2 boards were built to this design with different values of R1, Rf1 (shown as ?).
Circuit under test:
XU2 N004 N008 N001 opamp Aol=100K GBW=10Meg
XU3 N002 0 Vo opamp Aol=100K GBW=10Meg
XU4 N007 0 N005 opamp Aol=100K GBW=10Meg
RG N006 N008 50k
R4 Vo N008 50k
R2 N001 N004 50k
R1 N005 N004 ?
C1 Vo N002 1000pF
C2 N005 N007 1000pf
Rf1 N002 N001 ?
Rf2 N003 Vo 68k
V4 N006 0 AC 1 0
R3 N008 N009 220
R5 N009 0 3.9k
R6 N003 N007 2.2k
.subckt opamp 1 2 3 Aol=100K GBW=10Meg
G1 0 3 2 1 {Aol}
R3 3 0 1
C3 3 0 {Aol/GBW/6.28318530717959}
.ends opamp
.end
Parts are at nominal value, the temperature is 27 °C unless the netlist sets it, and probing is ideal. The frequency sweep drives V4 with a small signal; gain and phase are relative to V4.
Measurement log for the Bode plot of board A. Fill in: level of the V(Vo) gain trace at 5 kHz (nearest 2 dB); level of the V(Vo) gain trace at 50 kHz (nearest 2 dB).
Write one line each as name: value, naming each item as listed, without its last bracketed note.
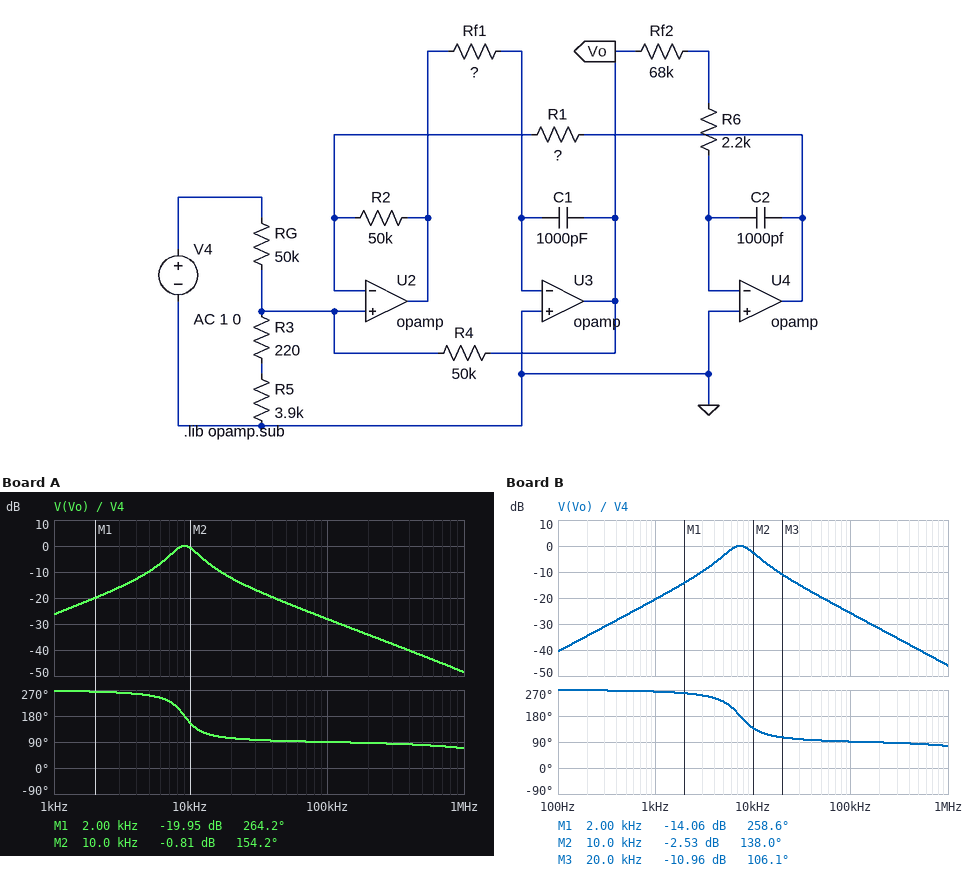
level of the V(Vo) gain trace at 5 kHz: -10 dB
level of the V(Vo) gain trace at 50 kHz: -22 dB
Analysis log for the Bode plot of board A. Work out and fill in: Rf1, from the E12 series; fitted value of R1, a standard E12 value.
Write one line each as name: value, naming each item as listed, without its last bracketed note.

Rf1, from the E12 series: 8.2 kΩ
fitted value of R1, a standard E12 value: 27 kΩ
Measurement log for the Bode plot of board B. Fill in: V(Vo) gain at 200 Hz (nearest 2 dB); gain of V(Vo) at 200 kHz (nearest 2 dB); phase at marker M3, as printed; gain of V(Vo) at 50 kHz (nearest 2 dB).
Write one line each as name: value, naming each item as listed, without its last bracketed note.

V(Vo) gain at 200 Hz: -34 dB
gain of V(Vo) at 200 kHz: -32 dB
phase at marker M3, as printed: 106.1 deg
gain of V(Vo) at 50 kHz: -20 dB
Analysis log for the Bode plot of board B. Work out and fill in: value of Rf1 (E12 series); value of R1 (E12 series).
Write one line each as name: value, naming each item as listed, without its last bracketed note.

value of Rf1: 3.3 kΩ
value of R1: 100 kΩ
